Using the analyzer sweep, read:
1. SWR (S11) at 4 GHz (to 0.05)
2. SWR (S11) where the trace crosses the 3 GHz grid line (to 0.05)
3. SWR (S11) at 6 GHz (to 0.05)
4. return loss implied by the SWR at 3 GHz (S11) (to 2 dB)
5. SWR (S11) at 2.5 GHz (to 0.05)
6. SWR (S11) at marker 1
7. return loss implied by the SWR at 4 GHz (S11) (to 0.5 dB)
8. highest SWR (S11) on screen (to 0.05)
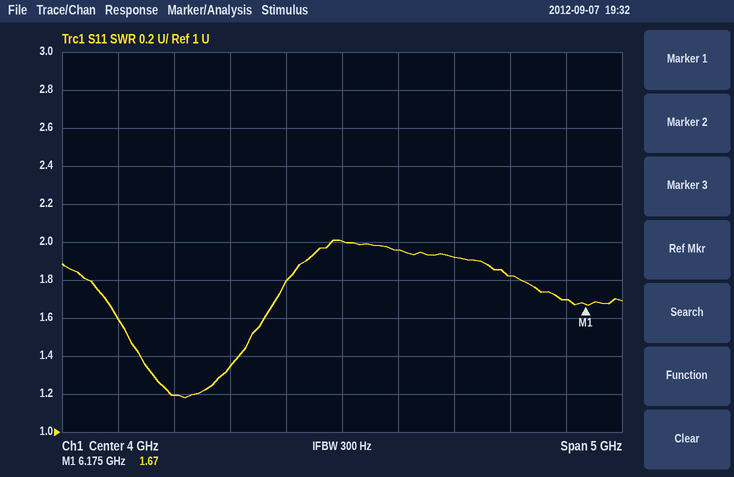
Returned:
2.00
1.35
1.70
16 dB
1.20
1.67
9.5 dB
2.00
